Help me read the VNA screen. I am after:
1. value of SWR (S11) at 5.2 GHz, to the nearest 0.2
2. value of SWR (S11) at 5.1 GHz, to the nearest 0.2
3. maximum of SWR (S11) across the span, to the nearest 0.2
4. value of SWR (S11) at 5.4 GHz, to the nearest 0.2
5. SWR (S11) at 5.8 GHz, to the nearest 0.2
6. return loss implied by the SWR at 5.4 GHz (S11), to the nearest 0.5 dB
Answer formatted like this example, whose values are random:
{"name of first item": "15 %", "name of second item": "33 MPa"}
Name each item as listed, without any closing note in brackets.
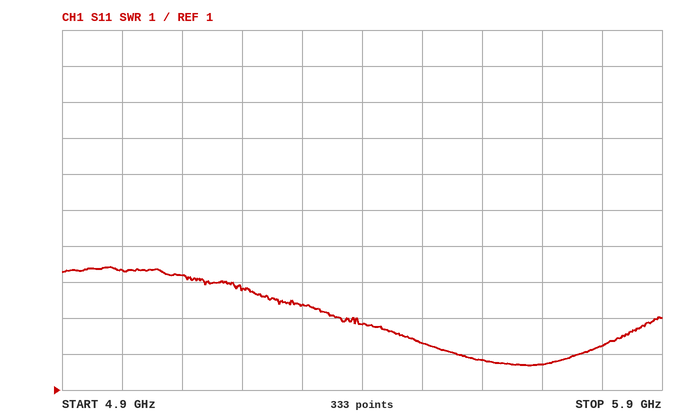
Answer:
{"value of SWR (S11) at 5.2 GHz, to the nearest 0.2": "3.8", "value of SWR (S11) at 5.1 GHz, to the nearest 0.2": "4.2", "maximum of SWR (S11) across the span, to the nearest 0.2": "4.4", "value of SWR (S11) at 5.4 GHz, to the nearest 0.2": "2.8", "SWR (S11) at 5.8 GHz, to the nearest 0.2": "2.2", "return loss implied by the SWR at 5.4 GHz (S11), to the nearest 0.5 dB": "6.5 dB"}
